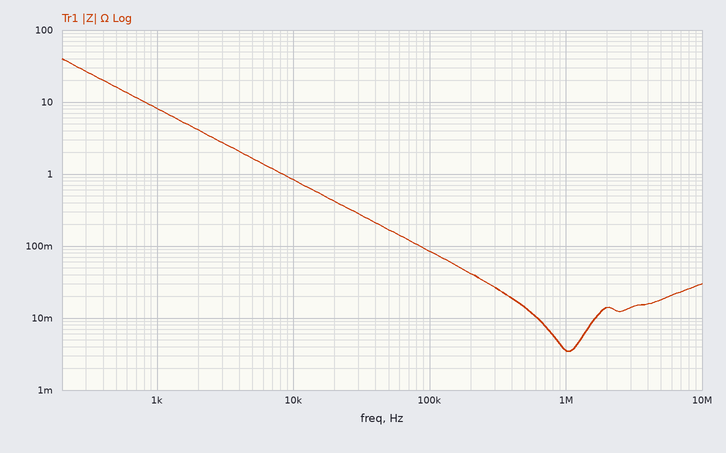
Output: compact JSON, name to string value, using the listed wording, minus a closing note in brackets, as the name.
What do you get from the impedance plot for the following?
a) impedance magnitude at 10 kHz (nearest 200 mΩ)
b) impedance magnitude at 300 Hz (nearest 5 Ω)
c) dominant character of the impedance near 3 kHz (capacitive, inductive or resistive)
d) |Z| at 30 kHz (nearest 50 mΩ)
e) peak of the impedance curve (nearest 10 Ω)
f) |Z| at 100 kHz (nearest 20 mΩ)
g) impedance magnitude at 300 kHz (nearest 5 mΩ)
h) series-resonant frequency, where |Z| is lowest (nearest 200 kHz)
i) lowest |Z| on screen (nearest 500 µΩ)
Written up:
{"impedance magnitude at 10 kHz": "800 mΩ", "impedance magnitude at 300 Hz": "25 Ω", "dominant character of the impedance near 3 kHz": "capacitive", "|Z| at 30 kHz": "300 mΩ", "peak of the impedance curve": "40 Ω", "|Z| at 100 kHz": "80 mΩ", "impedance magnitude at 300 kHz": "25 mΩ", "series-resonant frequency, where |Z| is lowest": "1.0 MHz", "lowest |Z| on screen": "3.5 mΩ"}
